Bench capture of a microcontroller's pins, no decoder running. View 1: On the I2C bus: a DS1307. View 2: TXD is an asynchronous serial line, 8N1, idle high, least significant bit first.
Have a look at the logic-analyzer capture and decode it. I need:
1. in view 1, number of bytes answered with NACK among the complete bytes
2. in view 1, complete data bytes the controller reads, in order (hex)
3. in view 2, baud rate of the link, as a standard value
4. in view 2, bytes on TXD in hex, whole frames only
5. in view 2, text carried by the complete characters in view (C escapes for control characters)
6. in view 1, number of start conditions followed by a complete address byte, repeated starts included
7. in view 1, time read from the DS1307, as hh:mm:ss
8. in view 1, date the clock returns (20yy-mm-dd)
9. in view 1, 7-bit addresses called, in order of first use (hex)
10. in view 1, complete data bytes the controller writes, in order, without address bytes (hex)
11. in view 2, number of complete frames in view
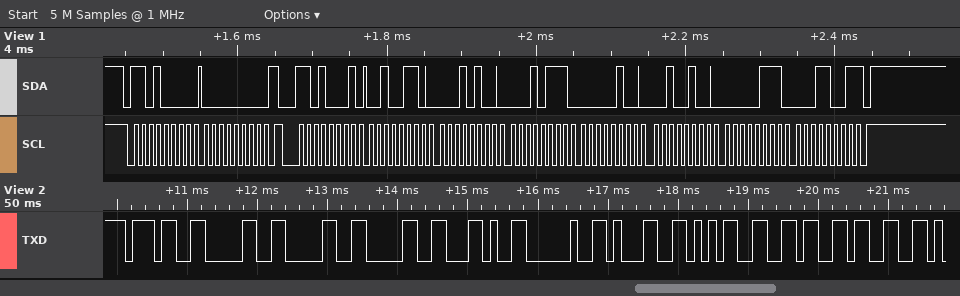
1
26 14 17 04 24 07 19
9600 baud
37 30 30 30 2C 20 31 35 36 33
"7000, 1563"
2
17:14:26
2019-07-24
0x68
00
10
